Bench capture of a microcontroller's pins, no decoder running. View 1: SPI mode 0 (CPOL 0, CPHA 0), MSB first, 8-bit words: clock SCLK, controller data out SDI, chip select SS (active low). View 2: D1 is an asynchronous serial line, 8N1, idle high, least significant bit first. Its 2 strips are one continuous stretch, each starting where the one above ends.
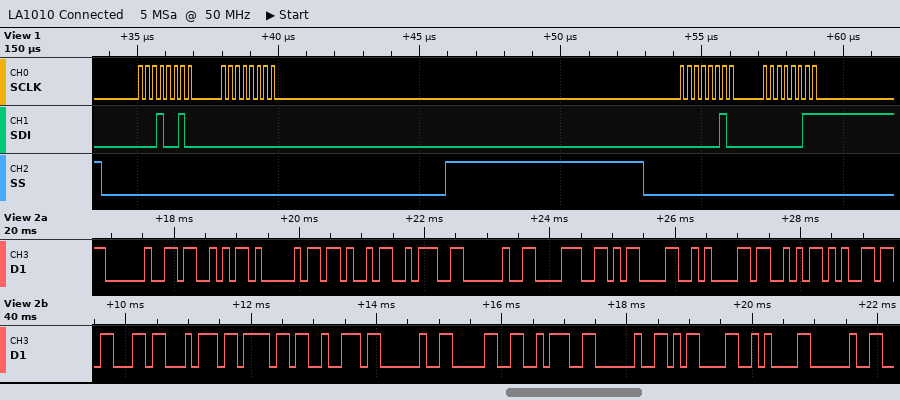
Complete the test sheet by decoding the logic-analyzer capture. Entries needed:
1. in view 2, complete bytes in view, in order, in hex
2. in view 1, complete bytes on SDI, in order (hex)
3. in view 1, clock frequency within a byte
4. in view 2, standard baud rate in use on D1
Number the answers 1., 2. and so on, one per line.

1. 0x20 0x53 0x41 0x4B 0x3A 0x20 0x38 0x0D 0x0A 0x53 0x65 0x63 0x74 0x6F 0x72 0x20 0x30 0x3A 0x20 0x0D 0x0A 0x20
2. 0x12 0x00 0x02 0x03
3. 4 MHz
4. 9600 baud
